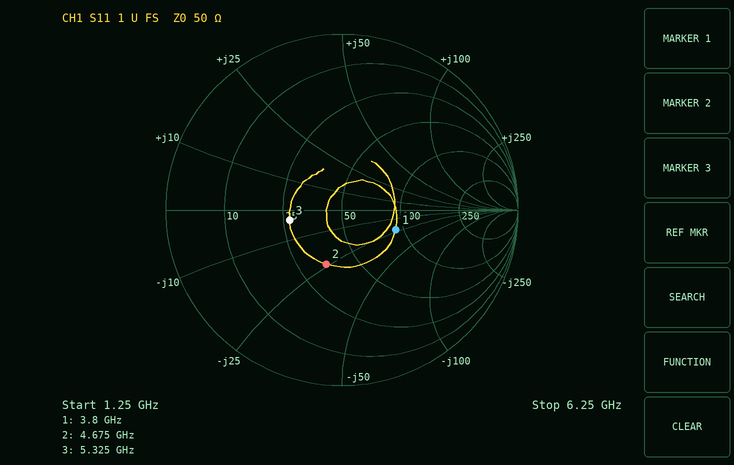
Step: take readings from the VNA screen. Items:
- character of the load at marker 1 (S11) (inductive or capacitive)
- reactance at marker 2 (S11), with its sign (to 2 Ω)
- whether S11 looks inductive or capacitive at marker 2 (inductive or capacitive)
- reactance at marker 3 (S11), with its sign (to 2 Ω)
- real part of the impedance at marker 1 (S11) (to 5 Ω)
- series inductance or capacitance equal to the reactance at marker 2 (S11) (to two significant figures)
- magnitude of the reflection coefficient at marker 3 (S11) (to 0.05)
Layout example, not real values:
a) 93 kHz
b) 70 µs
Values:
a) capacitive
b) -24 Ω
c) capacitive
d) -4 Ω
e) 90 Ω
f) 1.4 pF
g) 0.30
